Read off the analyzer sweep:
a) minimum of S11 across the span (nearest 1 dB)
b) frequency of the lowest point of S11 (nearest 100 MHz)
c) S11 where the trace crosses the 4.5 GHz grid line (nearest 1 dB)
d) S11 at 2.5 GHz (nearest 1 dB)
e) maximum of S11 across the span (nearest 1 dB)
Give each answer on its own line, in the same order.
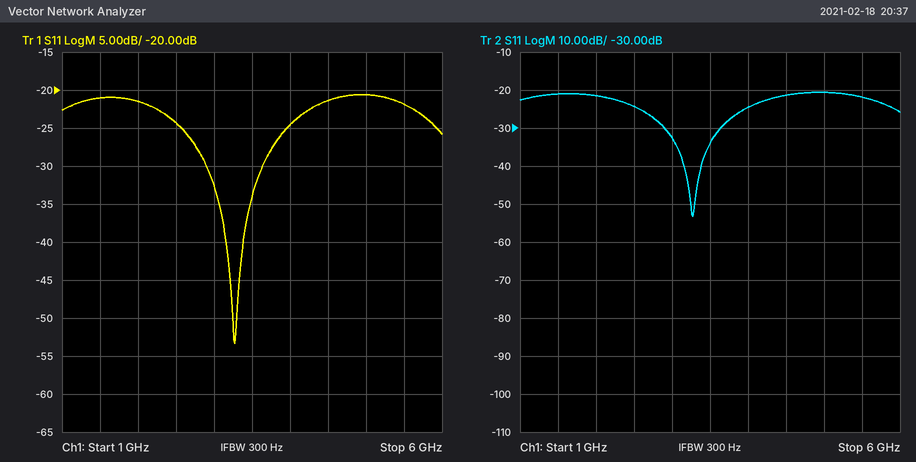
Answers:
-53 dB
3.3 GHz
-21 dB
-24 dB
-21 dB
